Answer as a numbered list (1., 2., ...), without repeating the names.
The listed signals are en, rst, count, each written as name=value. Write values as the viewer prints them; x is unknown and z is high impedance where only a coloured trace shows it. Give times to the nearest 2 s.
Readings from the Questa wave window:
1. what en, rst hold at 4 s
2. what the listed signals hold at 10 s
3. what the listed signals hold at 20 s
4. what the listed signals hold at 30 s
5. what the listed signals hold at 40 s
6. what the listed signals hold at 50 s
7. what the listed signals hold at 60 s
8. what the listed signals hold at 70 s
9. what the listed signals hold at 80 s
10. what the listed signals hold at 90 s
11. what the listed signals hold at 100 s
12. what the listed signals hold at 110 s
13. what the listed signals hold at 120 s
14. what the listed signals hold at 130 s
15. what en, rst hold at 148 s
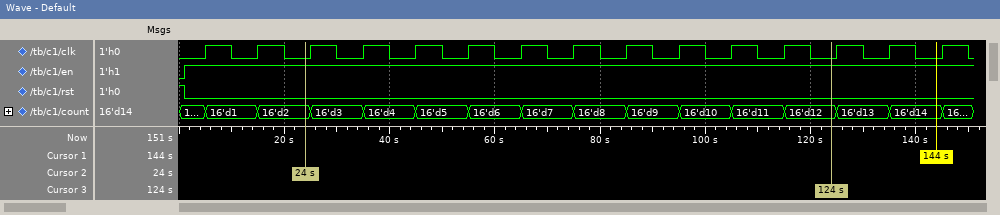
1. en=1, rst=0
2. en=1, rst=0, count=16'd1
3. en=1, rst=0, count=16'd2
4. en=1, rst=0, count=16'd3
5. en=1, rst=0, count=16'd4
6. en=1, rst=0, count=16'd5
7. en=1, rst=0, count=16'd6
8. en=1, rst=0, count=16'd7
9. en=1, rst=0, count=16'd8
10. en=1, rst=0, count=16'd9
11. en=1, rst=0, count=16'd10
12. en=1, rst=0, count=16'd11
13. en=1, rst=0, count=16'd12
14. en=1, rst=0, count=16'd13
15. en=1, rst=0
